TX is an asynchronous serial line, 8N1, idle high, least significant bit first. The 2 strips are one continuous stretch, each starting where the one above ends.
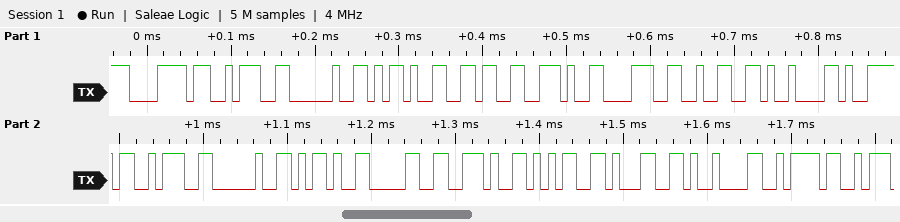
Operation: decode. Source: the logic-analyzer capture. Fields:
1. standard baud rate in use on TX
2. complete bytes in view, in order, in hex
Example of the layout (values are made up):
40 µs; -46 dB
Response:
115200 baud; 0x78 0x3A 0x20 0x2D 0x36 0x2E 0x38 0x32 0x09 0x79 0x3A 0x20 0x2D 0x30 0x2E 0x35 0x31 0x09 0x7A
